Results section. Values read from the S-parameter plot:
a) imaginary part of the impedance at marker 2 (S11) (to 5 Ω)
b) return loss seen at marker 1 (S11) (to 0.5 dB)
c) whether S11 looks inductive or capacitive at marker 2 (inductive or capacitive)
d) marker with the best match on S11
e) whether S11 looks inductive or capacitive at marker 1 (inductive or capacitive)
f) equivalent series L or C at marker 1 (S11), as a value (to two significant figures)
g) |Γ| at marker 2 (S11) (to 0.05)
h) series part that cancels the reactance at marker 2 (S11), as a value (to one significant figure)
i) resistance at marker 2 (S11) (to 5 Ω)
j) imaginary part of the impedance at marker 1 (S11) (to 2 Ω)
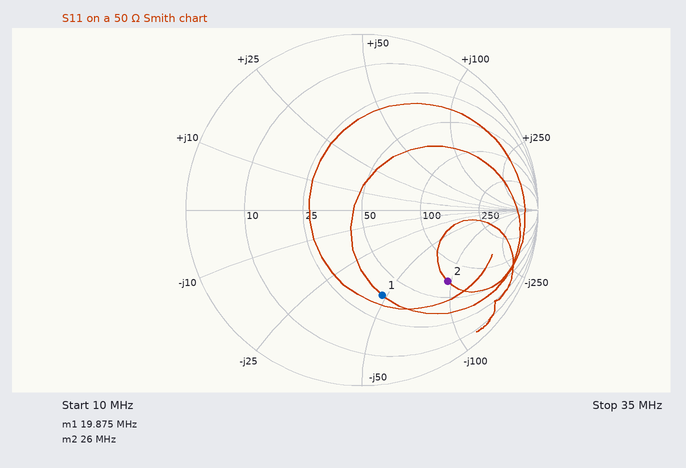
-95 Ω
6.0 dB
capacitive
marker 1
capacitive
170 pF
0.65
600 nH
70 Ω
-48 Ω
